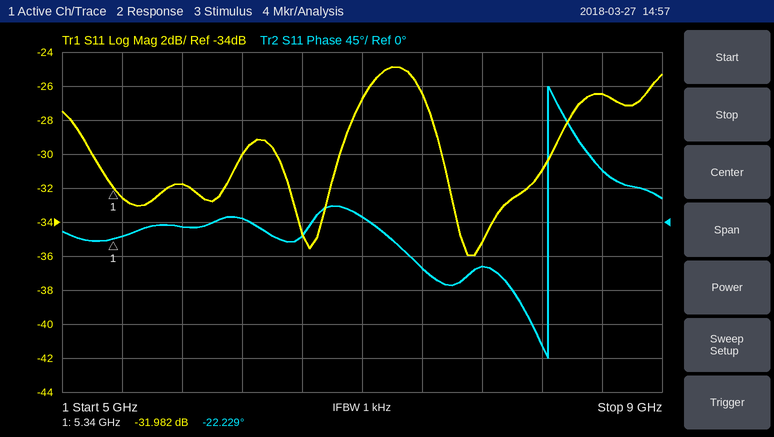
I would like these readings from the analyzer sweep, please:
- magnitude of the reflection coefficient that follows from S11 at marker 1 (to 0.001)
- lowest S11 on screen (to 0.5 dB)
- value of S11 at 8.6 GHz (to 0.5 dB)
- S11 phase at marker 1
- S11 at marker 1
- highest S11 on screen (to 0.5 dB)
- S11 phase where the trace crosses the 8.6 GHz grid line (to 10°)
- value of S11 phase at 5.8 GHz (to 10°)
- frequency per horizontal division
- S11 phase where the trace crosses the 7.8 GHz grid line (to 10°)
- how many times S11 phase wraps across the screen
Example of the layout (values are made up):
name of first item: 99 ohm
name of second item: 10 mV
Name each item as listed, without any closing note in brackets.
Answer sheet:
magnitude of the reflection coefficient that follows from S11 at marker 1: 0.025
lowest S11 on screen: -36.0 dB
value of S11 at 8.6 GHz: -26.5 dB
S11 phase at marker 1: -22.229°
S11 at marker 1: -31.982 dB
highest S11 on screen: -25.0 dB
S11 phase where the trace crosses the 8.6 GHz grid line: 70°
value of S11 phase at 5.8 GHz: -10°
frequency per horizontal division: 400 MHz
S11 phase where the trace crosses the 7.8 GHz grid line: -60°
how many times S11 phase wraps across the screen: 1
